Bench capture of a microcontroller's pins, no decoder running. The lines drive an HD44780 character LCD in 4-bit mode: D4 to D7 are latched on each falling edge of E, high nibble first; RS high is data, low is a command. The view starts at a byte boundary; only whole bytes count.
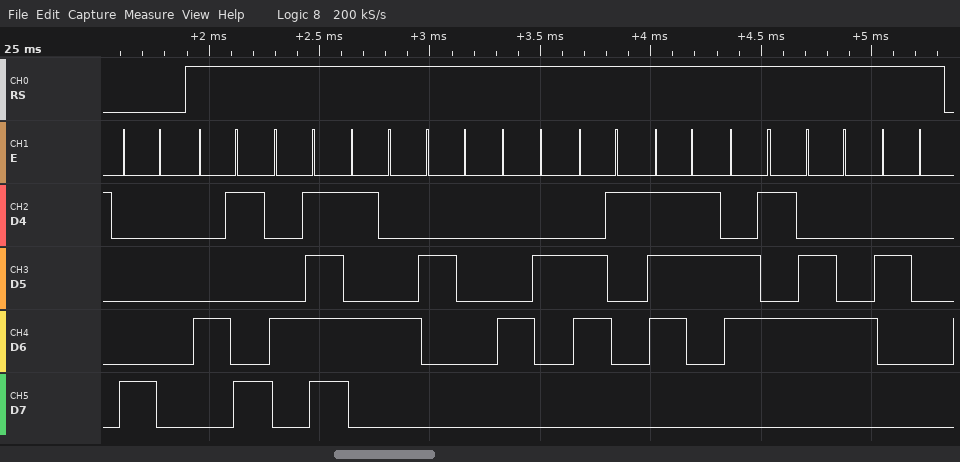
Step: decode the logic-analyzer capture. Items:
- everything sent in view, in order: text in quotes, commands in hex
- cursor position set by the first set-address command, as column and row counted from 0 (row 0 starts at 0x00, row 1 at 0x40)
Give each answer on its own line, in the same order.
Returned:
0x80 "IOT Based "
column 0, row 0
